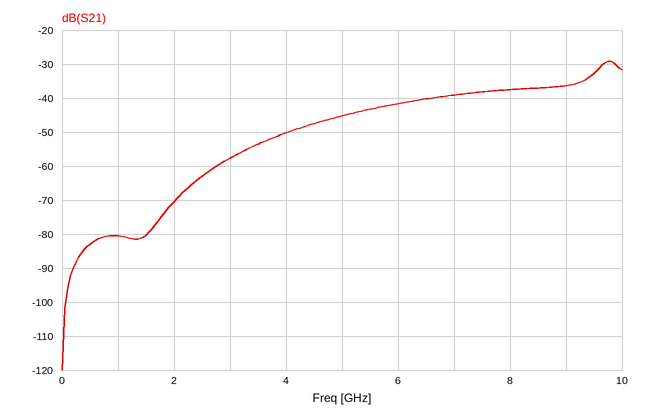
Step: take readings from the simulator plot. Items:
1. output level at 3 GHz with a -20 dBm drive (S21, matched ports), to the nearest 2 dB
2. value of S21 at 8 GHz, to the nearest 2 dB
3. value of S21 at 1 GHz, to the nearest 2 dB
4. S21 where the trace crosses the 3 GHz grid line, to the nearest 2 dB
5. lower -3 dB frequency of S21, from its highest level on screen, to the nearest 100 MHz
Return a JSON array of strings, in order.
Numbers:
["-78 dBm", "-38 dB", "-80 dB", "-58 dB", "9.5 GHz"]
